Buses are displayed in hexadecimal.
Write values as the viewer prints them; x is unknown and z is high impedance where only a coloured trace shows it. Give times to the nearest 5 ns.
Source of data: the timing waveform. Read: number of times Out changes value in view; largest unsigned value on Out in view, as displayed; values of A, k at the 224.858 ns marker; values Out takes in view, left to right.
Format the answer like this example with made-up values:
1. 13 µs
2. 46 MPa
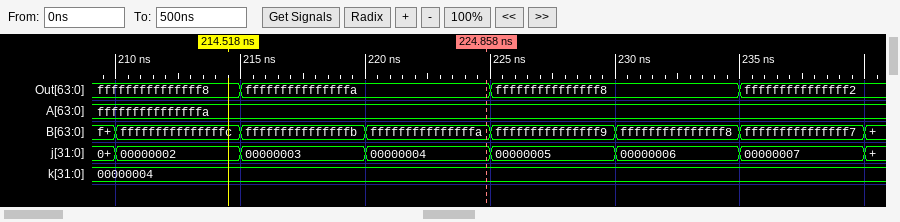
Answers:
1. 3
2. fffffffffffffffa
3. A=fffffffffffffffa, k=00000004
4. fffffffffffffff8, fffffffffffffffa, fffffffffffffff8, fffffffffffffff2
